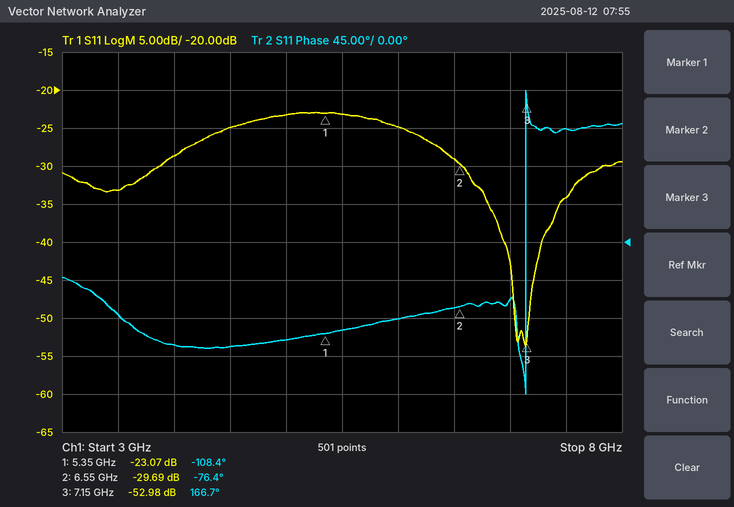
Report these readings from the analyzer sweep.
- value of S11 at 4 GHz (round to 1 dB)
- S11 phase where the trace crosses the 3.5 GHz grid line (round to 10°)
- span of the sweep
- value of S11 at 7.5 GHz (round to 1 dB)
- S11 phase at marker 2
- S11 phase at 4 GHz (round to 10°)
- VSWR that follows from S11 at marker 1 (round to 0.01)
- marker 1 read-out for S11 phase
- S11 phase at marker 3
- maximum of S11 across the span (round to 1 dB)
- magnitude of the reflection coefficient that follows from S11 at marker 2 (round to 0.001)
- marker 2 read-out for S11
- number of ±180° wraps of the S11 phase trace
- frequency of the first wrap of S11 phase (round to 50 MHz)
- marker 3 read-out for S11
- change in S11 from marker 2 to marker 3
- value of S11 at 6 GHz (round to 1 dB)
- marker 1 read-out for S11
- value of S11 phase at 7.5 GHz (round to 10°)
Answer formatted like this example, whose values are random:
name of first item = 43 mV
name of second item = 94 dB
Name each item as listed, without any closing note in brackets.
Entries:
value of S11 at 4 GHz = -29 dB
S11 phase where the trace crosses the 3.5 GHz grid line = -90°
span of the sweep = 5 GHz
value of S11 at 7.5 GHz = -34 dB
S11 phase at marker 2 = -76.4°
S11 phase at 4 GHz = -120°
VSWR that follows from S11 at marker 1 = 1.15
marker 1 read-out for S11 phase = -108.4°
S11 phase at marker 3 = 166.7°
maximum of S11 across the span = -23 dB
magnitude of the reflection coefficient that follows from S11 at marker 2 = 0.033
marker 2 read-out for S11 = -29.69 dB
number of ±180° wraps of the S11 phase trace = 1
frequency of the first wrap of S11 phase = 7.15 GHz
marker 3 read-out for S11 = -52.98 dB
change in S11 from marker 2 to marker 3 = -23.29 dB
value of S11 at 6 GHz = -25 dB
marker 1 read-out for S11 = -23.07 dB
value of S11 phase at 7.5 GHz = 130°
